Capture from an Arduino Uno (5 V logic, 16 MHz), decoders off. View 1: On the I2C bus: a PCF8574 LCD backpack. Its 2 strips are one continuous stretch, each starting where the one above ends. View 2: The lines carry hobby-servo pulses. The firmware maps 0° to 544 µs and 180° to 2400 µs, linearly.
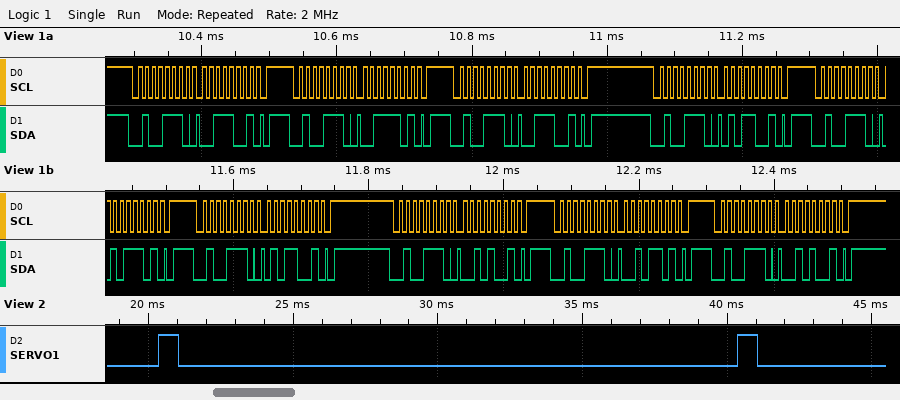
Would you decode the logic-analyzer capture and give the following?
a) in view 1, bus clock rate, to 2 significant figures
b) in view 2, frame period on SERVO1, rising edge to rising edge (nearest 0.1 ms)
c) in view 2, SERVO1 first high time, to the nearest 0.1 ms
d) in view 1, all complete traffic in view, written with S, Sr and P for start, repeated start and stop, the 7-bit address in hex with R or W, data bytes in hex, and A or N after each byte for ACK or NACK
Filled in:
100 kHz
20.0 ms
0.7 ms
S 27W A 39 A P S 27W A 3D A P S 27W A 39 A P S 27W A 59 A P S 27W A 5D A P S 27W A 59 A P S 27W A 29 A P S 27W A 2D A P S 27W A 29 A P
